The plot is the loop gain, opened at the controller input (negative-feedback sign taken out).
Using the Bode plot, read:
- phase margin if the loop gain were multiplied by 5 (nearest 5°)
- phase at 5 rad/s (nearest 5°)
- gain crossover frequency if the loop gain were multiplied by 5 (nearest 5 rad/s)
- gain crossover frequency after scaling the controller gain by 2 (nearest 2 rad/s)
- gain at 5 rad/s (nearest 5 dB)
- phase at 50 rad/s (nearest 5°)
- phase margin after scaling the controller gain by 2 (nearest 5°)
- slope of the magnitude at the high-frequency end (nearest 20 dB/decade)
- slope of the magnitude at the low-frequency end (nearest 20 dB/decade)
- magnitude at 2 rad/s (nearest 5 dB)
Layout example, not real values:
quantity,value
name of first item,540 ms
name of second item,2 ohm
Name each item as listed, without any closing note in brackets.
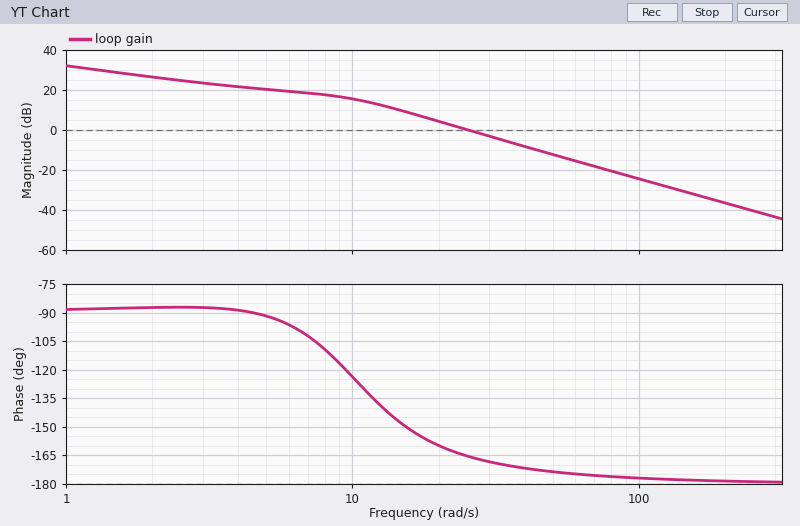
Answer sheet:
quantity,value
phase margin if the loop gain were multiplied by 5,5°
phase at 5 rad/s,-90°
gain crossover frequency if the loop gain were multiplied by 5,55 rad/s
gain crossover frequency after scaling the controller gain by 2,36 rad/s
gain at 5 rad/s,20 dB
phase at 50 rad/s,-175°
phase margin after scaling the controller gain by 2,10°
slope of the magnitude at the high-frequency end,-40 dB/decade
slope of the magnitude at the low-frequency end,-20 dB/decade
magnitude at 2 rad/s,25 dB
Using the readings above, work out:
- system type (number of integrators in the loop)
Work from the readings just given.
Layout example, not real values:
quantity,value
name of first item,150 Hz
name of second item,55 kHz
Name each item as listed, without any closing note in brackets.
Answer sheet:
quantity,value
system type,1
